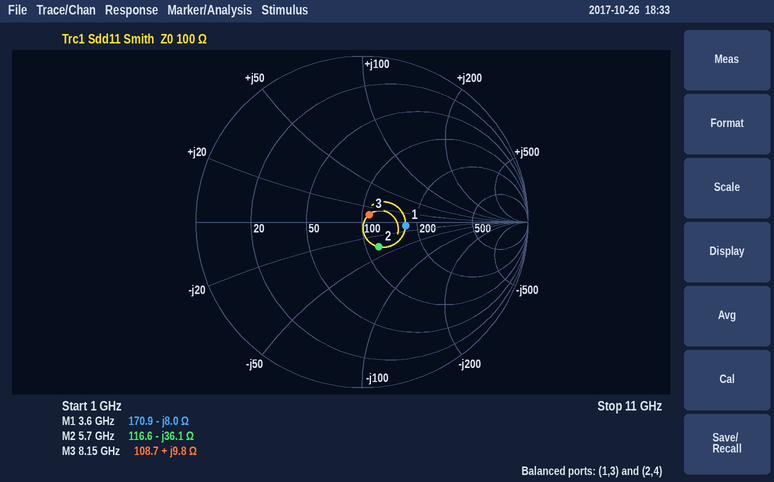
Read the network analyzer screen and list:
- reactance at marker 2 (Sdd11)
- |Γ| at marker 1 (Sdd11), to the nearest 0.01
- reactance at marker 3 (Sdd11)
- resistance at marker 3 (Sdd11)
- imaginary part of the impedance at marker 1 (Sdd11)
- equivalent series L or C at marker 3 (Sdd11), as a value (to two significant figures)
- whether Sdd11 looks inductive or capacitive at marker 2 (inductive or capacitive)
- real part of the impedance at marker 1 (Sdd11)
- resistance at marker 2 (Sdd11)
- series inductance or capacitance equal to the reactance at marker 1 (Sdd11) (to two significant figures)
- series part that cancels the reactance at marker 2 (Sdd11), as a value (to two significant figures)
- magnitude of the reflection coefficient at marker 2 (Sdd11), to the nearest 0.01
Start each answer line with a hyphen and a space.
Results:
- -36.1 Ω
- 0.26
- +9.8 Ω
- 108.7 Ω
- -8.0 Ω
- 190 pH
- capacitive
- 170.9 Ω
- 116.6 Ω
- 5.5 pF
- 1.0 nH
- 0.18
